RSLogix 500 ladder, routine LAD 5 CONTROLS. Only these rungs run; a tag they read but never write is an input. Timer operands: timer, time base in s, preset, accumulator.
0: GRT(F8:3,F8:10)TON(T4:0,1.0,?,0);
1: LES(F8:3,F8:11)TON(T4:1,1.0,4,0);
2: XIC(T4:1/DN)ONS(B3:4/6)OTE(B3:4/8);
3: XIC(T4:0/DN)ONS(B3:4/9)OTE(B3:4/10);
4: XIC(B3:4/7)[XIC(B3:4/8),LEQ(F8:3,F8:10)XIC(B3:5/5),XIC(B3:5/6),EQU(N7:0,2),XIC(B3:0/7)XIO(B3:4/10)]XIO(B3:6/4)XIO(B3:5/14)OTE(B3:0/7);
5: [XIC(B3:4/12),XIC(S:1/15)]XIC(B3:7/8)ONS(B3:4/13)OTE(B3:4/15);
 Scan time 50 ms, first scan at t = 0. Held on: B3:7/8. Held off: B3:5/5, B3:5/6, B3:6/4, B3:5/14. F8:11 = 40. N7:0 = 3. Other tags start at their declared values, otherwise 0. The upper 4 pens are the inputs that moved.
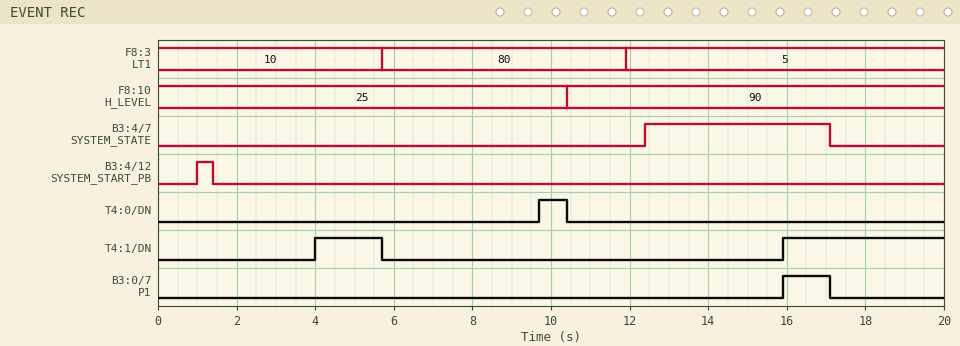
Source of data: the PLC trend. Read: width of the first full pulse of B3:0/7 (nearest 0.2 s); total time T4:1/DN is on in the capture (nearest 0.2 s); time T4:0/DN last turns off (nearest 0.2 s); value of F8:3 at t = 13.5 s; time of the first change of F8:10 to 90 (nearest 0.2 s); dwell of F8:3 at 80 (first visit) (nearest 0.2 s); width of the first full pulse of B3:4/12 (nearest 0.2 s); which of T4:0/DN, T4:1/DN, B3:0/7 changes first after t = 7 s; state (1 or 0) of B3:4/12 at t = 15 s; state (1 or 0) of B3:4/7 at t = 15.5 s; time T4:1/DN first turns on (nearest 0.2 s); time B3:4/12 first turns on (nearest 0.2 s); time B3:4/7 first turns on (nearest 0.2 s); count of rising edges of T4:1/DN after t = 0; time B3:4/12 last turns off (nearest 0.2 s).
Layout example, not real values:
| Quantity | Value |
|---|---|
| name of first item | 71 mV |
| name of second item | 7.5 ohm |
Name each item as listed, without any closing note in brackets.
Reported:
| Quantity | Value |
|---|---|
| width of the first full pulse of B3:0/7 | 1.2 s |
| total time T4:1/DN is on in the capture | 5.8 s |
| time T4:0/DN last turns off | 10.4 s |
| value of F8:3 at t = 13.5 s | 5 |
| time of the first change of F8:10 to 90 | 10.4 s |
| dwell of F8:3 at 80 (first visit) | 6.2 s |
| width of the first full pulse of B3:4/12 | 0.4 s |
| which of T4:0/DN, T4:1/DN, B3:0/7 changes first after t = 7 s | T4:0/DN |
| state (1 or 0) of B3:4/12 at t = 15 s | 0 |
| state (1 or 0) of B3:4/7 at t = 15.5 s | 1 |
| time T4:1/DN first turns on | 4.0 s |
| time B3:4/12 first turns on | 1.0 s |
| time B3:4/7 first turns on | 12.4 s |
| count of rising edges of T4:1/DN after t = 0 | 2 |
| time B3:4/12 last turns off | 1.4 s |
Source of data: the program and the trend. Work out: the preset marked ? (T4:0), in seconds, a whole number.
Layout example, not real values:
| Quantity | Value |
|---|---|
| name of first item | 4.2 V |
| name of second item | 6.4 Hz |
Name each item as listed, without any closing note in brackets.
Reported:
| Quantity | Value |
|---|---|
| the preset marked ? (T4:0), in seconds, a whole number | 4 s |
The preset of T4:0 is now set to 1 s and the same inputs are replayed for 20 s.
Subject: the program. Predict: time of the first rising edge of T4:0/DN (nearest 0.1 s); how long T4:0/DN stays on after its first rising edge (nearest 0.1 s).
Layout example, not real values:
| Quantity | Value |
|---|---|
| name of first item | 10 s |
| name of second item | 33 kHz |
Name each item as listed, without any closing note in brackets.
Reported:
| Quantity | Value |
|---|---|
| time of the first rising edge of T4:0/DN | 6.7 s |
| how long T4:0/DN stays on after its first rising edge | 3.7 s |
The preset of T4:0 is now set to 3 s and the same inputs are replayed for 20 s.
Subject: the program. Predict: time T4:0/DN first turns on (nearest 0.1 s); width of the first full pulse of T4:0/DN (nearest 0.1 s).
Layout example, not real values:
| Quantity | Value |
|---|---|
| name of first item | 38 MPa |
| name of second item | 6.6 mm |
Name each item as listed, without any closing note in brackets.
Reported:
| Quantity | Value |
|---|---|
| time T4:0/DN first turns on | 8.7 s |
| width of the first full pulse of T4:0/DN | 1.7 s |
